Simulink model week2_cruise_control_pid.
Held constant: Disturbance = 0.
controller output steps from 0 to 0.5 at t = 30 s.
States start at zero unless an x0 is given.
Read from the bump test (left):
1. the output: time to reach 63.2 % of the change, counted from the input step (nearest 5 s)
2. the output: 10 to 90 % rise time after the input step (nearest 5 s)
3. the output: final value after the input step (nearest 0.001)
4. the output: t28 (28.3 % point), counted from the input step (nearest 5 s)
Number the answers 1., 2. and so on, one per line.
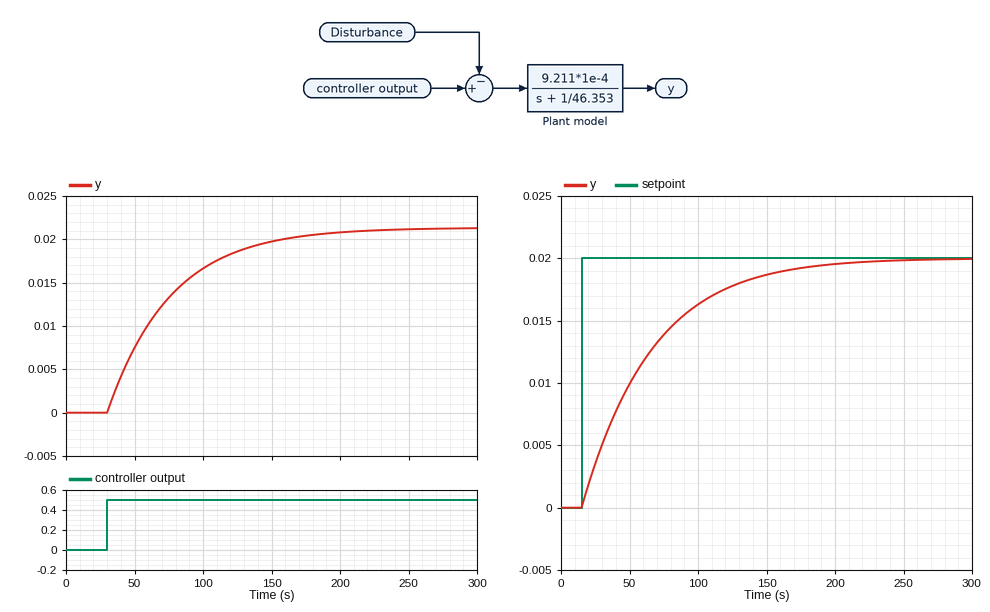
1. 45 s
2. 100 s
3. 0.021
4. 15 s
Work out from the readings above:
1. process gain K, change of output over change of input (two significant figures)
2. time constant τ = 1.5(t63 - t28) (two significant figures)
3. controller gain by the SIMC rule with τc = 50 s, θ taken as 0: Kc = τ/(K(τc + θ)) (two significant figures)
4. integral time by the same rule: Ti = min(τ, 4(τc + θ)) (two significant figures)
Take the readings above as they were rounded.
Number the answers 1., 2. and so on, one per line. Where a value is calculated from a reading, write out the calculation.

1. (0.021 - 0) / 0.5 = 0.042
2. 1.5 × (45 - 15) = 45 s
3. 45 / (0.042 × (50 + 0)) = 21
4. min(45, 4 × (50 + 0)) = 45 s
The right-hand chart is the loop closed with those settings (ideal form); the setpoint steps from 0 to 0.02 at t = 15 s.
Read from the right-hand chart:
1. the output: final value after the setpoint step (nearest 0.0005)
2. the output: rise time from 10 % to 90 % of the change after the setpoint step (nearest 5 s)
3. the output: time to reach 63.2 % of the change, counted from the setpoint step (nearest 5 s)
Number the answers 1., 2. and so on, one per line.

1. 0.0200
2. 110 s
3. 50 s
